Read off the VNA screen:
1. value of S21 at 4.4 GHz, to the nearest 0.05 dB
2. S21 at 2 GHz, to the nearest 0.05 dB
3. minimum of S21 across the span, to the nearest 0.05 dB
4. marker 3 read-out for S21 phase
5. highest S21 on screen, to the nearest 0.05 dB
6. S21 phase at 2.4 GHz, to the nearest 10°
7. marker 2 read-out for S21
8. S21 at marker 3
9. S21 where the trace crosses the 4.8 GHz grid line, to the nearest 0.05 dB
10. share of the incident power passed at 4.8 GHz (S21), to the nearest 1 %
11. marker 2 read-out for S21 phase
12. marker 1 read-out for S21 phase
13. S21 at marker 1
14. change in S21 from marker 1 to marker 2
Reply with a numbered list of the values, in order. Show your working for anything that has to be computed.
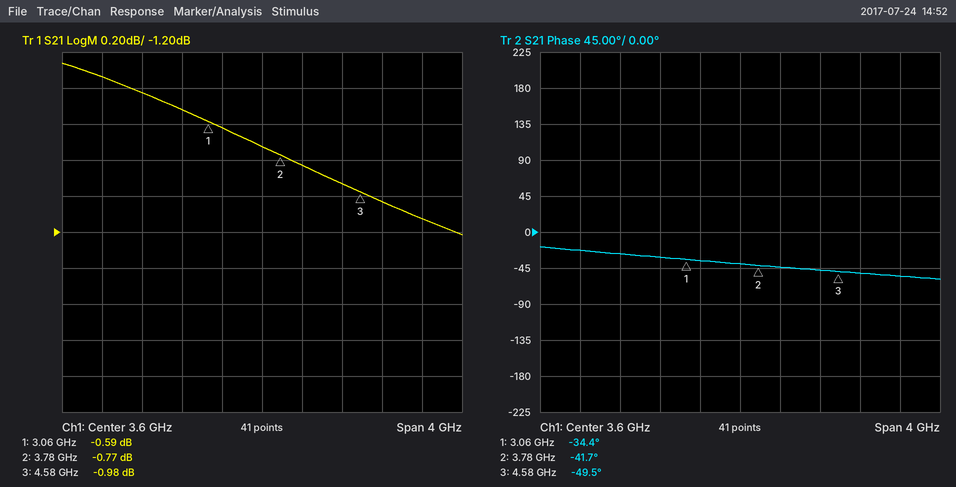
1. -0.95 dB
2. -0.35 dB
3. -1.20 dB
4. -49.5°
5. -0.25 dB
6. -30°
7. -0.77 dB
8. -0.98 dB
9. -1.05 dB
10. 10^(-1.05/10) ≈ 79 %
11. -41.7°
12. -34.4°
13. -0.59 dB
14. -0.77 − (-0.59) = -0.18 dB
